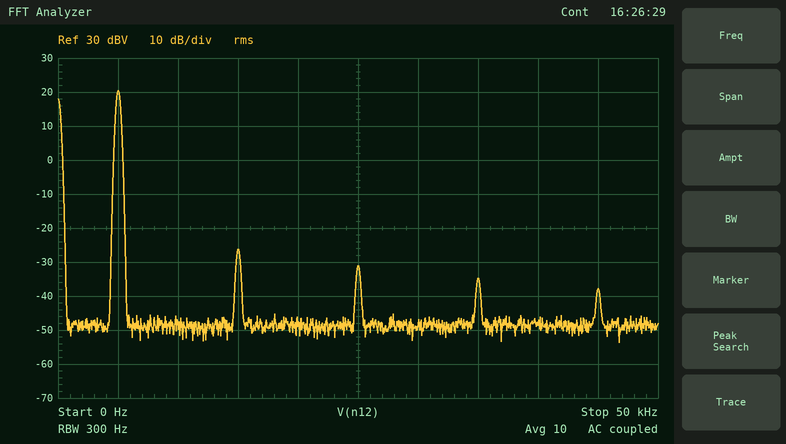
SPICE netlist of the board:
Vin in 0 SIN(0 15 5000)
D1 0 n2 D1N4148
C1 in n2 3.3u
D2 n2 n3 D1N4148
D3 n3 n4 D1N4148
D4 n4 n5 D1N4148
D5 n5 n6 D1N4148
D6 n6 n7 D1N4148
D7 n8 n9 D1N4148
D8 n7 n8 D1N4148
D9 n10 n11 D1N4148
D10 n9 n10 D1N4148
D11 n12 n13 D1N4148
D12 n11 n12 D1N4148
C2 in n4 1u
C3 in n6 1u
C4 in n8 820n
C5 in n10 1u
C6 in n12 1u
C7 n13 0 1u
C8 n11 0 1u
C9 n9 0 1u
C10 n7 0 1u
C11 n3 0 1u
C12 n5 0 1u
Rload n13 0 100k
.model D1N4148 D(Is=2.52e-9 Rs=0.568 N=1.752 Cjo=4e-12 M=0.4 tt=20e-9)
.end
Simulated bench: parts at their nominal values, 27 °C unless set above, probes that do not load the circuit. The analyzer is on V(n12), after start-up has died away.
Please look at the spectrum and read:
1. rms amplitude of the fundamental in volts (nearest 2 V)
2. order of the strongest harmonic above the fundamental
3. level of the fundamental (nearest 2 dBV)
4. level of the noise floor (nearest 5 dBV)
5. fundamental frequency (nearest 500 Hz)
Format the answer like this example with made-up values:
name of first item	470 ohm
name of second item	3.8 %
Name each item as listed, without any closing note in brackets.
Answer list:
rms amplitude of the fundamental in volts	10 V
order of the strongest harmonic above the fundamental	3
level of the fundamental	20 dBV
level of the noise floor	-50 dBV
fundamental frequency	5.0 kHz
